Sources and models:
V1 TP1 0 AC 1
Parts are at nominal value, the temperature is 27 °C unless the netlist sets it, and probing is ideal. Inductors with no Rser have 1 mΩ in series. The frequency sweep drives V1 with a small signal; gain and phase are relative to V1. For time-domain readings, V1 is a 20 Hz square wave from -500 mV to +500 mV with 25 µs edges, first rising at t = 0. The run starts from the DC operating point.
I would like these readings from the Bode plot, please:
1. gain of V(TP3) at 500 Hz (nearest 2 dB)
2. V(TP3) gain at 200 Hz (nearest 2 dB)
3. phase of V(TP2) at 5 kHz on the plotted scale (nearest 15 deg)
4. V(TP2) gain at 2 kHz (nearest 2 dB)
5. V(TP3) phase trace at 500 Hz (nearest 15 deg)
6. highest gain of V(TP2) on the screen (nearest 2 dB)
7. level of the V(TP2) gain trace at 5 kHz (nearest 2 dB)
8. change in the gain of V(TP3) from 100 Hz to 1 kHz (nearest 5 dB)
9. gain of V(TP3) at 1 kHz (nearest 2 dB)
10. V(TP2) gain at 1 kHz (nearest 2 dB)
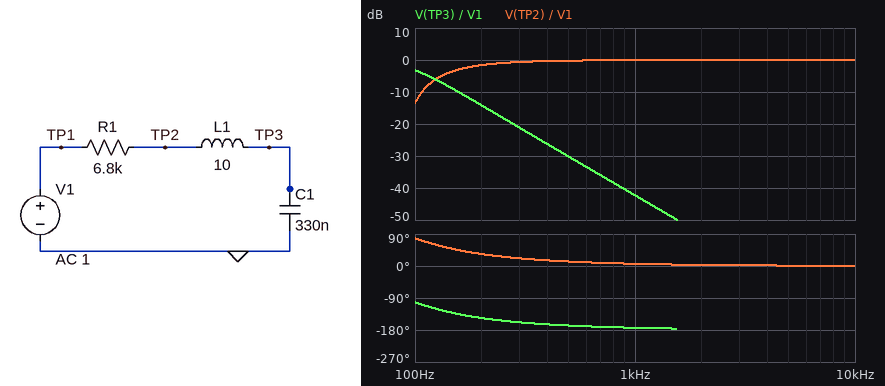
-30 dB
-14 dB
0 deg
0 dB
-165 deg
0 dB
0 dB
-40 dB
-42 dB
0 dB
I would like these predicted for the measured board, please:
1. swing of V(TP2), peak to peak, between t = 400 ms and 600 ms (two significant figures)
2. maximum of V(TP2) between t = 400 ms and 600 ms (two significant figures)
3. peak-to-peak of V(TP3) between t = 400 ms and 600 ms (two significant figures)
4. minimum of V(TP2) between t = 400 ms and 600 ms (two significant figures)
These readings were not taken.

1.1 V
550 mV
1.2 V
-550 mV
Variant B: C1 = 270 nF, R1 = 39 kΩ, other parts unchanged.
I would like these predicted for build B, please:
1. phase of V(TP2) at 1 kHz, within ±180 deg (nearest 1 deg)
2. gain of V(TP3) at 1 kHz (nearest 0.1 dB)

32 deg
-41.9 dB
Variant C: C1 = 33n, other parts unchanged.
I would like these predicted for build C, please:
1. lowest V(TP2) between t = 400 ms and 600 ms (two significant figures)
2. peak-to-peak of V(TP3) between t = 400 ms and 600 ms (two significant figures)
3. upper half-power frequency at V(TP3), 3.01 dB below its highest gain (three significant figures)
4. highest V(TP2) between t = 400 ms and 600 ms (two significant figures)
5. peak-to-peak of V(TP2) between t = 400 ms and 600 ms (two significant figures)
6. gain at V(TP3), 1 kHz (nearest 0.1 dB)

-660 mV
2.1 V
317 Hz
660 mV
1.3 V
-21.7 dB
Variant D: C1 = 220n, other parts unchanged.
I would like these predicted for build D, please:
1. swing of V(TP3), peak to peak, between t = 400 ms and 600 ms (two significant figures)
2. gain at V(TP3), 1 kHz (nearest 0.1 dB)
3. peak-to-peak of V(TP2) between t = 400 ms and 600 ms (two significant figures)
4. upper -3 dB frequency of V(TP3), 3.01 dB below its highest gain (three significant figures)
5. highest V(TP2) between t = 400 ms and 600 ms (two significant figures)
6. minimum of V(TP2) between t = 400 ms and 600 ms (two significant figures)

1.3 V
-38.7 dB
1.2 V
125 Hz
590 mV
-590 mV
